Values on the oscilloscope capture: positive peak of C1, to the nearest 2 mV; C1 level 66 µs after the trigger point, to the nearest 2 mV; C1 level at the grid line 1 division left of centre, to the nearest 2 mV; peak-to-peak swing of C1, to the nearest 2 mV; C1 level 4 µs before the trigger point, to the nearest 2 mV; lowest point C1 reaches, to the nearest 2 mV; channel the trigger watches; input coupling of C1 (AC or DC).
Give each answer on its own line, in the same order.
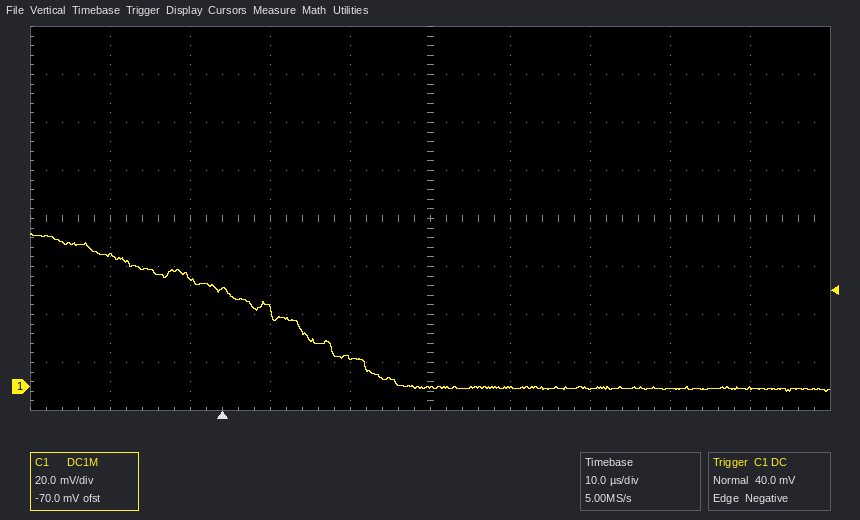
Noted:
64 mV
0 mV
12 mV
66 mV
46 mV
-2 mV
C1
DC
